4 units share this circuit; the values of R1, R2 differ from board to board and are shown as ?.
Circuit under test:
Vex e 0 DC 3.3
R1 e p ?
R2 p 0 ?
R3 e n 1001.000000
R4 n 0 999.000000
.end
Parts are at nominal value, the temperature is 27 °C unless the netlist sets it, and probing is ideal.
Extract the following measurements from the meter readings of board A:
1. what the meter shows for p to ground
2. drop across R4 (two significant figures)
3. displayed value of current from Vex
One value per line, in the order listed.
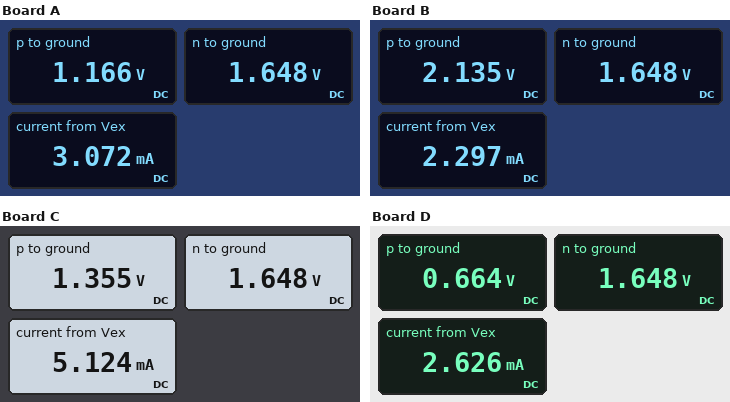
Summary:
1.166 V
1.6 V
3.072 mA
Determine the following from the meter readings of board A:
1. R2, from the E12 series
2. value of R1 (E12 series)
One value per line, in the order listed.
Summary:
820 Ω
1.5 kΩ
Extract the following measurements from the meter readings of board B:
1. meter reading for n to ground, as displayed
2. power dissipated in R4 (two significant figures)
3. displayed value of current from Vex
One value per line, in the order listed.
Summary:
1.648 V
2.7 mW
2.297 mA
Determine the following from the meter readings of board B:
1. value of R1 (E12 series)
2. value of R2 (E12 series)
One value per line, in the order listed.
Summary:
1.8 kΩ
3.3 kΩ
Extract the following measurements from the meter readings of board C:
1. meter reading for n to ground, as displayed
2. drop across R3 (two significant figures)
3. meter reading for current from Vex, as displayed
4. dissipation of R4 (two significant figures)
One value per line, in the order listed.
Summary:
1.648 V
1.7 V
5.124 mA
2.7 mW
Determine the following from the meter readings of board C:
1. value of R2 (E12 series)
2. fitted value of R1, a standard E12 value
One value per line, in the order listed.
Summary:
390 Ω
560 Ω
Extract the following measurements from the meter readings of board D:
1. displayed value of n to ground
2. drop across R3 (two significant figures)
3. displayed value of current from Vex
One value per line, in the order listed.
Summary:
1.648 V
1.7 V
2.626 mA
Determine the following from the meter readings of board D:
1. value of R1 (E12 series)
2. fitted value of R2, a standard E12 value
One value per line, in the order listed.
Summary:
2.7 kΩ
680 Ω
